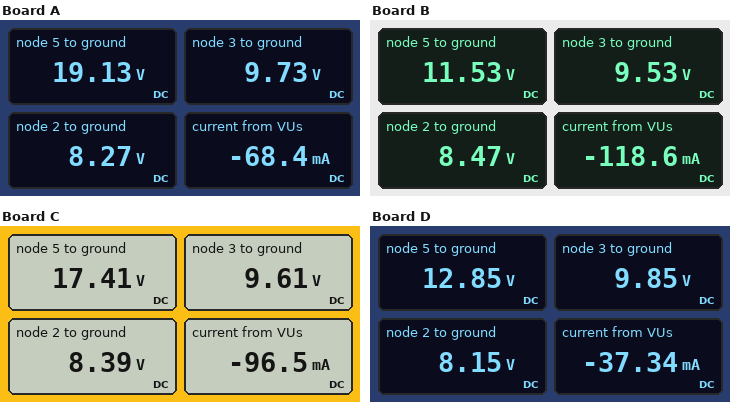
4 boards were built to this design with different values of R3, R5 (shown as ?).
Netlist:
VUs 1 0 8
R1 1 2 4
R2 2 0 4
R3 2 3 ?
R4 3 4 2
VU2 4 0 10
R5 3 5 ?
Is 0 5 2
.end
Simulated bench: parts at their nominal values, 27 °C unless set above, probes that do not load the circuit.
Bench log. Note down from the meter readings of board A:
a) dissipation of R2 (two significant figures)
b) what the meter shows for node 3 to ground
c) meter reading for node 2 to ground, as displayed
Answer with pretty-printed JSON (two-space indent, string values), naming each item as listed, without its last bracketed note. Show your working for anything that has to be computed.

{
  "dissipation of R2": "(8.27 V)^2 / 4 Ω = 17 W",
  "what the meter shows for node 3 to ground": "9.73 V",
  "meter reading for node 2 to ground, as displayed": "8.27 V"
}
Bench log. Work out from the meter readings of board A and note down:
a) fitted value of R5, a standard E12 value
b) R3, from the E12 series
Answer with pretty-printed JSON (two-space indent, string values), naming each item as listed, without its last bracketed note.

{
  "fitted value of R5, a standard E12 value": "4.7 Ω",
  "R3, from the E12 series": "0.68 Ω"
}
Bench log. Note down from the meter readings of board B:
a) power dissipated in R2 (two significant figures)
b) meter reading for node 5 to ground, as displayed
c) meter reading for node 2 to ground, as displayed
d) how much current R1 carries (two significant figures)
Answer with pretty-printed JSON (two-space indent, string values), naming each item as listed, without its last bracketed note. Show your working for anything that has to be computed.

{
  "power dissipated in R2": "(8.47 V)^2 / 4 Ω = 18 W",
  "meter reading for node 5 to ground, as displayed": "11.53 V",
  "meter reading for node 2 to ground, as displayed": "8.47 V",
  "how much current R1 carries": "(8.47 V - 8 V) / 4 Ω = 120 mA"
}
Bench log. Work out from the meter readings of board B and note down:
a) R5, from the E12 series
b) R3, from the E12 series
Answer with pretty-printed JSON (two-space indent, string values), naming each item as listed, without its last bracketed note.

{
  "R5, from the E12 series": "1 Ω",
  "R3, from the E12 series": "0.47 Ω"
}
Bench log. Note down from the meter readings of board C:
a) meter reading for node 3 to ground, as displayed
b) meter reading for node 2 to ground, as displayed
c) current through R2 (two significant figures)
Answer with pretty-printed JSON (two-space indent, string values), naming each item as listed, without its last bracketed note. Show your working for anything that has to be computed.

{
  "meter reading for node 3 to ground, as displayed": "9.61 V",
  "meter reading for node 2 to ground, as displayed": "8.39 V",
  "current through R2": "(8.39 V) / 4 Ω = 2.1 A"
}
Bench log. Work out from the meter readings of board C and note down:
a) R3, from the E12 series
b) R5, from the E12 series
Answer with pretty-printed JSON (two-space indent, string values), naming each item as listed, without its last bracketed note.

{
  "R3, from the E12 series": "0.56 Ω",
  "R5, from the E12 series": "3.9 Ω"
}
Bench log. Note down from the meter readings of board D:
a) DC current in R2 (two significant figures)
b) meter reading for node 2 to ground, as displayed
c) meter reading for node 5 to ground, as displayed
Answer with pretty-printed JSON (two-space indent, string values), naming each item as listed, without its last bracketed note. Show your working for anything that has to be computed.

{
  "DC current in R2": "(8.15 V) / 4 Ω = 2.0 A",
  "meter reading for node 2 to ground, as displayed": "8.15 V",
  "meter reading for node 5 to ground, as displayed": "12.85 V"
}
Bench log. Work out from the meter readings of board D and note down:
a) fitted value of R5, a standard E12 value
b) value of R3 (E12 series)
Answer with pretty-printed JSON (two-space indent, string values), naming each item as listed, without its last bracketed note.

{
  "fitted value of R5, a standard E12 value": "1.5 Ω",
  "value of R3": "0.82 Ω"
}
